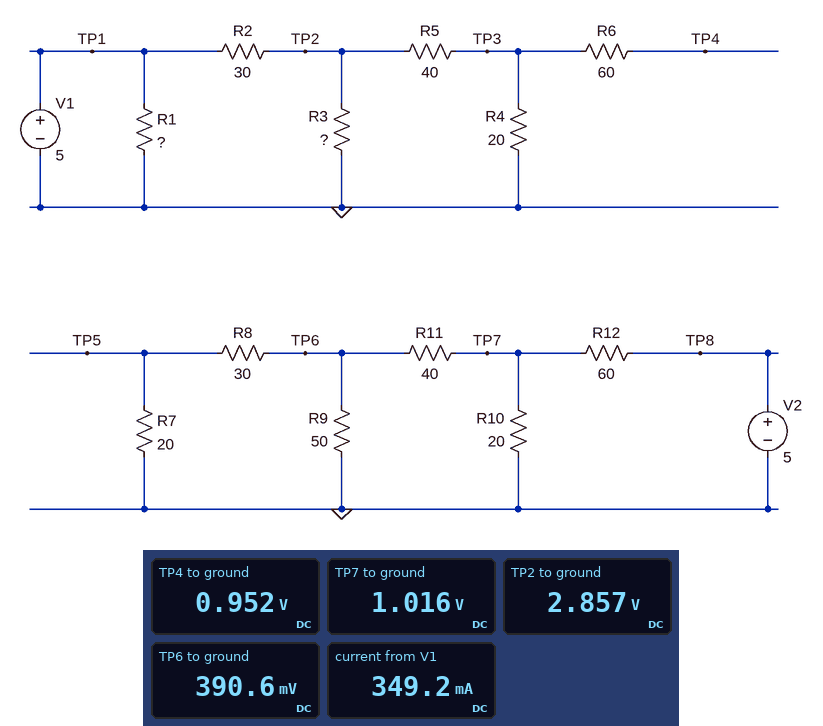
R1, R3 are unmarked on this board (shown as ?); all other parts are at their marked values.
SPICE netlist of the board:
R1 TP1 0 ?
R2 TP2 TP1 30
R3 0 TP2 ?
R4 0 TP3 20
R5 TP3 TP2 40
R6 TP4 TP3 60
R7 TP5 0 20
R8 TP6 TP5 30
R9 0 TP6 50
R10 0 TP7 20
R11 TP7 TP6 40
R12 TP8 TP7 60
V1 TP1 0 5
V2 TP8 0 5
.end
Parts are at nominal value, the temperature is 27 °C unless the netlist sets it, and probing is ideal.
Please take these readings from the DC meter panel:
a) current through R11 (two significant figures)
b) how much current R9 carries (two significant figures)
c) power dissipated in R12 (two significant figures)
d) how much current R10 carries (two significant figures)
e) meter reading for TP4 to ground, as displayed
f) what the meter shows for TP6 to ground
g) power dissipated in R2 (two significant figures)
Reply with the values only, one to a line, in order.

16 mA
7.8 mA
260 mW
51 mA
0.952 V
390.6 mV
150 mW
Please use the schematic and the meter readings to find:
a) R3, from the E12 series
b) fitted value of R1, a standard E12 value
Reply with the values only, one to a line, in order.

120 Ω
18 Ω
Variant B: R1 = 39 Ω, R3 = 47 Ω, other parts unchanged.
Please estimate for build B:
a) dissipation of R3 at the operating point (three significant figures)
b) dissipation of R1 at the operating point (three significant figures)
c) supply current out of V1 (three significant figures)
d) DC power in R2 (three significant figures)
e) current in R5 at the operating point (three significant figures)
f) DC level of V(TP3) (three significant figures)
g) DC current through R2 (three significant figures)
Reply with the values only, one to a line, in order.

116 mW
641 mW
217 mA
236 mW
39.0 mA
779 mV
88.7 mA
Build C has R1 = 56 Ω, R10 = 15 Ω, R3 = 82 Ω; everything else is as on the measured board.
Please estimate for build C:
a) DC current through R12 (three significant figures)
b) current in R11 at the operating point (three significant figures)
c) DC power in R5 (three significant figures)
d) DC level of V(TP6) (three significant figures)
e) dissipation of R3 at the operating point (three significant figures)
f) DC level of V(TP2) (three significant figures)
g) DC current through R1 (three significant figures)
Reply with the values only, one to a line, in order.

69.3 mA
13.0 mA
79.8 mW
325 mV
87.6 mW
2.68 V
89.3 mA
